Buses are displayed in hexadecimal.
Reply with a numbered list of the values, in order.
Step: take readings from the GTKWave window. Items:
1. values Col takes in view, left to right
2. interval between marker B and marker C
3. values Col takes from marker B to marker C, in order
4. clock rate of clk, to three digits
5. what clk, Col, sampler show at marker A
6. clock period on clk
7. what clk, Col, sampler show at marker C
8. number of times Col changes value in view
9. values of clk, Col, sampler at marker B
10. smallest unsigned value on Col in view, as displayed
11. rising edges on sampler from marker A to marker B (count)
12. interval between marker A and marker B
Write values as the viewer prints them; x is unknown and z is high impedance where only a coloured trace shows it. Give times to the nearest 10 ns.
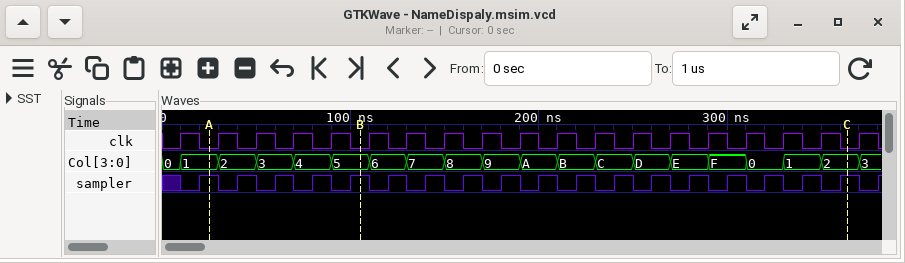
1. 0, 1, 2, 3, 4, 5, 6, 7, 8, 9, A, B, C, D, E, F, 0, 1, 2, 3
2. 260 ns
3. 5, 6, 7, 8, 9, A, B, C, D, E, F, 0, 1, 2
4. 50.0 MHz
5. clk=0, Col=1, sampler=1
6. 20 ns
7. clk=0, Col=2, sampler=1
8. 19
9. clk=0, Col=5, sampler=1
10. 0
11. 4
12. 80 ns
